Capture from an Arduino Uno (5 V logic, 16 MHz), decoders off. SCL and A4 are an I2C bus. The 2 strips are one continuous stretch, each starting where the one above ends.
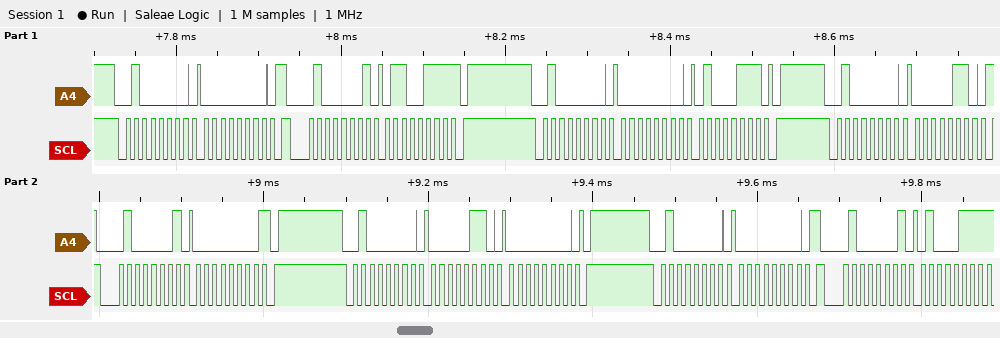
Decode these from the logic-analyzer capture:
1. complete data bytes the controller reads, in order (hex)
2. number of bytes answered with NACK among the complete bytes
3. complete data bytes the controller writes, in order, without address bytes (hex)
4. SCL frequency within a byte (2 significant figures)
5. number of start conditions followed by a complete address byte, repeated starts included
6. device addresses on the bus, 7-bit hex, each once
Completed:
67 00 47
3
00 00 47 06 06 00 00
100 kHz
8
0x20
